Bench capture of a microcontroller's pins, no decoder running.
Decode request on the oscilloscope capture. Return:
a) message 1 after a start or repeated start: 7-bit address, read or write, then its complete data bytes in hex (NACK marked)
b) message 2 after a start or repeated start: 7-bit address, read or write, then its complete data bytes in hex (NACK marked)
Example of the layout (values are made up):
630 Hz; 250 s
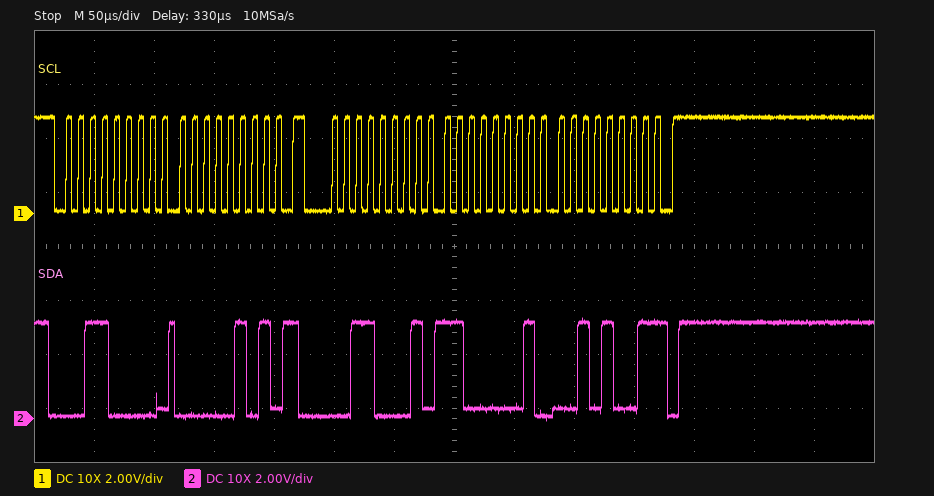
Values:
0x18 write: 05; 0x18 read: C1 29 NACK
